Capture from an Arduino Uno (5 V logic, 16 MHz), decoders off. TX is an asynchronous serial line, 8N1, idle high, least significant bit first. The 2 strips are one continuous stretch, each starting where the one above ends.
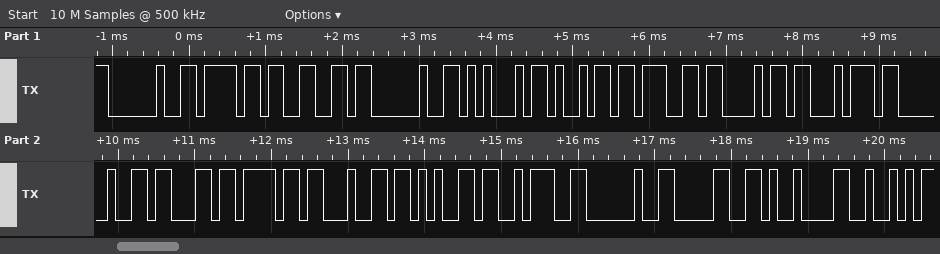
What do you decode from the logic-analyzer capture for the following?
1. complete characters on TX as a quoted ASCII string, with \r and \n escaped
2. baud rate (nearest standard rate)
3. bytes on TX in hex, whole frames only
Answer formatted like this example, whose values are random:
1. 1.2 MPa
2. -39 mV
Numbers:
1. " of Eight code: 0\tR"
2. 9600 baud
3. 0x20 0x6F 0x66 0x20 0x45 0x69 0x67 0x68 0x74 0x20 0x63 0x6F 0x64 0x65 0x3A 0x20 0x30 0x09 0x52
